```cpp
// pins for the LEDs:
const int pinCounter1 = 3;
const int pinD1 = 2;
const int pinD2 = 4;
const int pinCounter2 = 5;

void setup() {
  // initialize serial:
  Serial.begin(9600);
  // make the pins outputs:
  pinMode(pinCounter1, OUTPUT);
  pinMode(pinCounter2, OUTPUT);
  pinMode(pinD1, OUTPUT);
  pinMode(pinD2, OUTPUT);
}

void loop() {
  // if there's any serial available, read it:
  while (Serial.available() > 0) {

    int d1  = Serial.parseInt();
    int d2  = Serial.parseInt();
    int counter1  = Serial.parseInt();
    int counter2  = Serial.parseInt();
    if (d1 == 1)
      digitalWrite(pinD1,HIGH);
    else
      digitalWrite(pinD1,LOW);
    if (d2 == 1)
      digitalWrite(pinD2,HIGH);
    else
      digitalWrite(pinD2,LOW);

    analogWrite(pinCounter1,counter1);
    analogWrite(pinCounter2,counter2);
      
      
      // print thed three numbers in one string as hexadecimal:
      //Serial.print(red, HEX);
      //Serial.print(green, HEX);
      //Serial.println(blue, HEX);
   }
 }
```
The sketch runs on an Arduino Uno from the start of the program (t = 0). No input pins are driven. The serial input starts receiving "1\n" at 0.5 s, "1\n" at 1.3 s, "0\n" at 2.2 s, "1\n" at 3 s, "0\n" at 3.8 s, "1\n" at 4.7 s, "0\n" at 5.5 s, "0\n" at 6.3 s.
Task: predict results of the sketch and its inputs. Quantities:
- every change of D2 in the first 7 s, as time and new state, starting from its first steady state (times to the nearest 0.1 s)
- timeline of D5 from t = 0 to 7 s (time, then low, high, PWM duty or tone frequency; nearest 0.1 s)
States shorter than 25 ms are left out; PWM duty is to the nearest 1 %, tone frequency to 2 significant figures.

0 s low; 3 s high; 6.3 s low
0 s low; 3 s PWM 1 %; 6.3 s low
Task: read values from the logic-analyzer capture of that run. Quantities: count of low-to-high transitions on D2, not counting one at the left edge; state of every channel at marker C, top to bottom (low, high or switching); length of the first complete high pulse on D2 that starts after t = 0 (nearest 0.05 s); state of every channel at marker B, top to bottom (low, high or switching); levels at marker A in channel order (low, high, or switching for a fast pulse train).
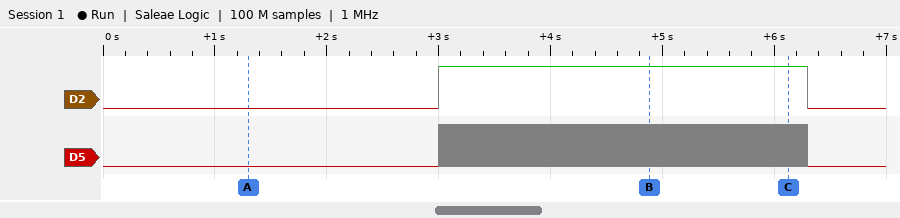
1
D2 high, D5 switching
3.30 s
D2 high, D5 switching
D2 low, D5 low
